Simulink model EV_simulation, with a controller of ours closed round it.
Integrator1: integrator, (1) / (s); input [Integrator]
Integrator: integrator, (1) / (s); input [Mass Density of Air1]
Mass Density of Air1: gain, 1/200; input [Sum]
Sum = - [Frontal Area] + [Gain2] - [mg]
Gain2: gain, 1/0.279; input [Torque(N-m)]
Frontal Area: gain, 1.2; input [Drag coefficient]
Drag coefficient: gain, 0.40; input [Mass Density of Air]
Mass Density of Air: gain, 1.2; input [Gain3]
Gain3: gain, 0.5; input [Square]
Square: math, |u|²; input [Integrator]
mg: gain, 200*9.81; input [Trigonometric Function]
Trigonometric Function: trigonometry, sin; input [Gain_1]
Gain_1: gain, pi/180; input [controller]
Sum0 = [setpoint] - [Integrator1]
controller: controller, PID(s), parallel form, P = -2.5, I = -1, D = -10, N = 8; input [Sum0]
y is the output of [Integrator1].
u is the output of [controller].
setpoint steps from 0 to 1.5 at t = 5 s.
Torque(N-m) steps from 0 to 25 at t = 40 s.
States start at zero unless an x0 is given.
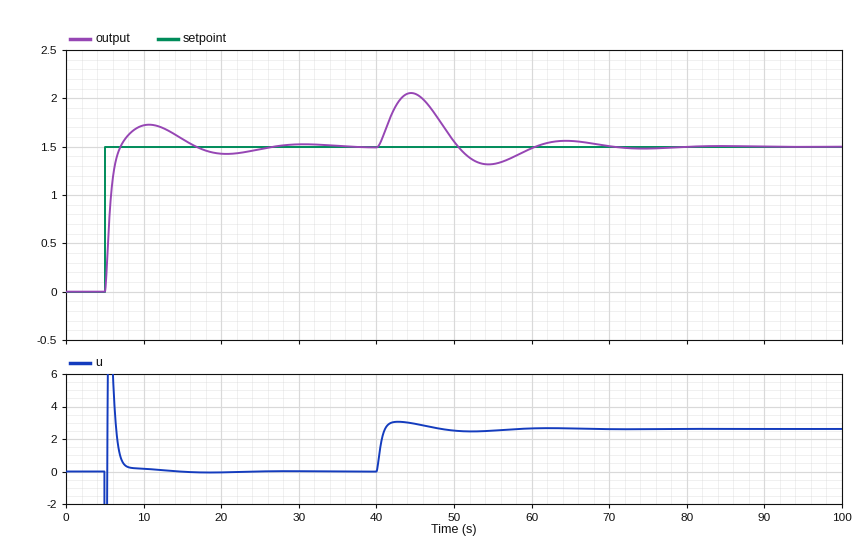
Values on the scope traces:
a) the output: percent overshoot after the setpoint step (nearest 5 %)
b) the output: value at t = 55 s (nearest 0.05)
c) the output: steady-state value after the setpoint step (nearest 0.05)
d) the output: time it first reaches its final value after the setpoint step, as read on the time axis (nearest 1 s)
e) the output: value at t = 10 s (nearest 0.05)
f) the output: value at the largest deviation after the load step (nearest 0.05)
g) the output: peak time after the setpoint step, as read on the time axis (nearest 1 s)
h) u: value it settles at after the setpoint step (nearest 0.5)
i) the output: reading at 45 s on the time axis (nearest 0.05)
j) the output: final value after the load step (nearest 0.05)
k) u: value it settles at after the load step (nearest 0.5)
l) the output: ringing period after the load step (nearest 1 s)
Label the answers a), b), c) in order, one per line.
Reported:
a) 15 %
b) 1.30
c) 1.50
d) 7 s
e) 1.70
f) 2.05
g) 11 s
h) 0.0
i) 2.05
j) 1.50
k) 2.5
l) 20 s
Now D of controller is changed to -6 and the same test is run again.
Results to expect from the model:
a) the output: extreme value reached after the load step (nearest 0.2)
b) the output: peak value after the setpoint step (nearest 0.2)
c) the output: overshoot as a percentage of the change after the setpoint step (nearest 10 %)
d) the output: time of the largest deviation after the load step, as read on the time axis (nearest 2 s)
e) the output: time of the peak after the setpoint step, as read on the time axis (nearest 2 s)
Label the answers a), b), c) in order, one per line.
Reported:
a) 2.2
b) 2.0
c) 30 %
d) 44 s
e) 8 s
